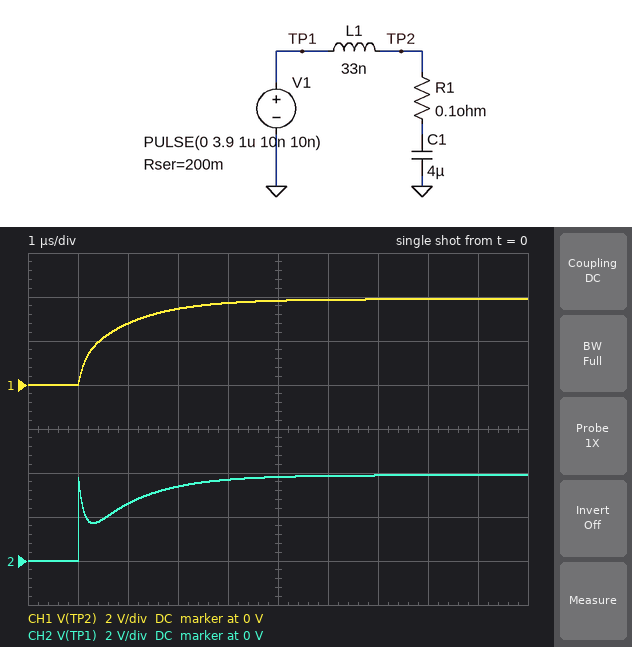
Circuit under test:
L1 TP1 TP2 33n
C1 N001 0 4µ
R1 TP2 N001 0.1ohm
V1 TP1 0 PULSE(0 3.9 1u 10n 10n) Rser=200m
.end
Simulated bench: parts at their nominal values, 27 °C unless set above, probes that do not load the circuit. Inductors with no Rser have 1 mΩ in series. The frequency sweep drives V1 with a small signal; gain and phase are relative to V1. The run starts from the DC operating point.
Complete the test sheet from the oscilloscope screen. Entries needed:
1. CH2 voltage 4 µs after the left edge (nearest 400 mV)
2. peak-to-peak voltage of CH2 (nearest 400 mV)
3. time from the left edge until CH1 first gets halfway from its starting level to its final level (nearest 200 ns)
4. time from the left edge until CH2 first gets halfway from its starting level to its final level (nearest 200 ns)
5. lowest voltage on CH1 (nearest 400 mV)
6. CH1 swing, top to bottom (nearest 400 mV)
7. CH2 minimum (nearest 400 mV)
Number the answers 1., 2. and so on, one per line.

1. 3.6 V
2. 4.0 V
3. 1.4 µs
4. 1.0 µs
5. 0 V
6. 4.0 V
7. 0 V
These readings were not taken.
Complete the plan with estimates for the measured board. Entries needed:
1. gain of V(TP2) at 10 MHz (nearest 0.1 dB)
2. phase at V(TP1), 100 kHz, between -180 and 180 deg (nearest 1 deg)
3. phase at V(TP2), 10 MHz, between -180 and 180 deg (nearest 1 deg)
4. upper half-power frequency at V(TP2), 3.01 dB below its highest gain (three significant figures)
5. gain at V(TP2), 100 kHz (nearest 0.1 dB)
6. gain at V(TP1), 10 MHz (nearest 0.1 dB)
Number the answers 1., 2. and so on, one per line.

1. -26.4 dB
2. -24 deg
3. -84 deg
4. 169 kHz
5. -1.4 dB
6. -0.1 dB
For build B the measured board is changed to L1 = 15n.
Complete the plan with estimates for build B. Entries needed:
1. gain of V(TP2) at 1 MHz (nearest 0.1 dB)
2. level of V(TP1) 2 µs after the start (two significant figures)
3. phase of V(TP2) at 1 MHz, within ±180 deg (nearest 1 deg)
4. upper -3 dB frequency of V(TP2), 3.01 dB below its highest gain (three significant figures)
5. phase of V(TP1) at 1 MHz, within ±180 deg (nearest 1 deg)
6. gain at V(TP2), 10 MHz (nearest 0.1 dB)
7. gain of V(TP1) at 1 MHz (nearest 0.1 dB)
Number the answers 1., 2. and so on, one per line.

1. -9.1 dB
2. 2.7 V
3. -32 deg
4. 158 kHz
5. 18 deg
6. -19.9 dB
7. -8.5 dB
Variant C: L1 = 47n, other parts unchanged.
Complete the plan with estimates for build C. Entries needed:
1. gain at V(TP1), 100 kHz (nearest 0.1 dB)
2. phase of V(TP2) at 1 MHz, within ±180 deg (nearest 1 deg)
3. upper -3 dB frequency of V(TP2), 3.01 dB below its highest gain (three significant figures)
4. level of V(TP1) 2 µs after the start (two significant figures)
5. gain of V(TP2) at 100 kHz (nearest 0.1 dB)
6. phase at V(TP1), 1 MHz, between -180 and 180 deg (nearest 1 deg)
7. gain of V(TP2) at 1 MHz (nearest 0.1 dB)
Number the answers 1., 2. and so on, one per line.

1. -1.9 dB
2. -62 deg
3. 178 kHz
4. 2.5 V
5. -1.3 dB
6. 28 deg
7. -11.3 dB
